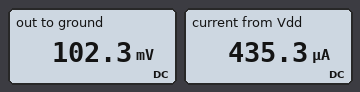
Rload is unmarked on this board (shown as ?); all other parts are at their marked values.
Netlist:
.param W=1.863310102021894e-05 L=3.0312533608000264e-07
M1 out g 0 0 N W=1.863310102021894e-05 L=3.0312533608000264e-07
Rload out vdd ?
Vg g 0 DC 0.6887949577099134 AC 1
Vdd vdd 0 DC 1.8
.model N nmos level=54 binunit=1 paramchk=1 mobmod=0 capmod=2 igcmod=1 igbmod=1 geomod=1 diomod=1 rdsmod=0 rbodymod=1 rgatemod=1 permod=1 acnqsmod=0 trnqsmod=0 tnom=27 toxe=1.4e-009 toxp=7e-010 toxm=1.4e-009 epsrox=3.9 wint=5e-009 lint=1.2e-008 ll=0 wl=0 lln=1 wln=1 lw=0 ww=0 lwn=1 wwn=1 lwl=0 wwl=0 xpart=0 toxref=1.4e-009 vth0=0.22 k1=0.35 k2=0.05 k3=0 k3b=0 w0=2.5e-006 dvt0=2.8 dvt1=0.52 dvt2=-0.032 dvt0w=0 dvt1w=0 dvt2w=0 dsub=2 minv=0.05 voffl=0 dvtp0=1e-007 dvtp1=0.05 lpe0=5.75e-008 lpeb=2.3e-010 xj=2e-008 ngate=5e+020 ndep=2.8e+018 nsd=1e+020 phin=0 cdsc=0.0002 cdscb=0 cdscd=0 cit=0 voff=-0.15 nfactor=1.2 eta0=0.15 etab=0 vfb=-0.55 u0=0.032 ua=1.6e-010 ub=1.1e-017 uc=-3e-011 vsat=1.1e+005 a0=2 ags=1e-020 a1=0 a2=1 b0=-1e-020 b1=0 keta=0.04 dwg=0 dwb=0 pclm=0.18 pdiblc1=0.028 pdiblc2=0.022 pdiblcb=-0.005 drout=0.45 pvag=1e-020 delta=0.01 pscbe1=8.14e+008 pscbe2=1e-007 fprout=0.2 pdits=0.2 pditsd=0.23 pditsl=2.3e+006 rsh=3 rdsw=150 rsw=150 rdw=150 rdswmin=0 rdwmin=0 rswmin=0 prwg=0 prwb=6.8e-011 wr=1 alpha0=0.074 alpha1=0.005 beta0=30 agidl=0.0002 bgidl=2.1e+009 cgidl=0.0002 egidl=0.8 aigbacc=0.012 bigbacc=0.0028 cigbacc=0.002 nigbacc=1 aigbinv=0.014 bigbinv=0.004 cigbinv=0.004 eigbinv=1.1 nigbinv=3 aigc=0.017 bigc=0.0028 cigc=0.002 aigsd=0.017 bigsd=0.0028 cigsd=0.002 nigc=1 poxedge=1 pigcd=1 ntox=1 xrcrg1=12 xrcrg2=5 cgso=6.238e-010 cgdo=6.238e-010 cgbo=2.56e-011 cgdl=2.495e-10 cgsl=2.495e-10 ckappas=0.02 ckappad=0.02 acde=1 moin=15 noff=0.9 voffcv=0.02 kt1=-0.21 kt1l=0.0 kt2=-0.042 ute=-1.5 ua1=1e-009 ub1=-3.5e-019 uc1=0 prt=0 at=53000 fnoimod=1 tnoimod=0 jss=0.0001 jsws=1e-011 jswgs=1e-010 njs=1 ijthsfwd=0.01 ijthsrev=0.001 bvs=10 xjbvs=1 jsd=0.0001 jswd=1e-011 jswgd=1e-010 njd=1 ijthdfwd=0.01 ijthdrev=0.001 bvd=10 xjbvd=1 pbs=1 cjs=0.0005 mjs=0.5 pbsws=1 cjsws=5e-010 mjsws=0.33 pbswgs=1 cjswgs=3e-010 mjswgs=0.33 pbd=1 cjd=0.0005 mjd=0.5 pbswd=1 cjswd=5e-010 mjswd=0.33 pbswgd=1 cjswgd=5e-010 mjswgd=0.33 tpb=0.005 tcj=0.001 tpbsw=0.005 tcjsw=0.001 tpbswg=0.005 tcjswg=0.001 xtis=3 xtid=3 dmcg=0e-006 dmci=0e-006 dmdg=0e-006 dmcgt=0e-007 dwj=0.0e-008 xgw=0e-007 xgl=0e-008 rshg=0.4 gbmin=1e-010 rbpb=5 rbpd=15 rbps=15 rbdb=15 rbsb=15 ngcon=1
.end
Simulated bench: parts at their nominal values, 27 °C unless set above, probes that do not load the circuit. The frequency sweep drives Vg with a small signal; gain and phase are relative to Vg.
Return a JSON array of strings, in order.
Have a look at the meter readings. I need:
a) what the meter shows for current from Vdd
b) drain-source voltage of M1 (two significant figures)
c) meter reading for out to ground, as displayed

["435.3 µA", "100 mV", "102.3 mV"]
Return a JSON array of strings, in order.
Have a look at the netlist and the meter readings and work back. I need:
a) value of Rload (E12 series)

["3.9 kΩ"]
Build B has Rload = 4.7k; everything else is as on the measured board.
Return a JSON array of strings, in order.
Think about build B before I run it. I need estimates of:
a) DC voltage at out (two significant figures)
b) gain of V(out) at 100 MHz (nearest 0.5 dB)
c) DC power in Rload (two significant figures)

["83 mV", "-18.5 dB", "630 µW"]
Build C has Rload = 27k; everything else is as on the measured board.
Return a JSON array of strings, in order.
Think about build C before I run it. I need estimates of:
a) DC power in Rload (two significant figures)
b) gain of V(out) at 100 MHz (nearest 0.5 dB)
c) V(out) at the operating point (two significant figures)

["120 µW", "-34.0 dB", "13 mV"]
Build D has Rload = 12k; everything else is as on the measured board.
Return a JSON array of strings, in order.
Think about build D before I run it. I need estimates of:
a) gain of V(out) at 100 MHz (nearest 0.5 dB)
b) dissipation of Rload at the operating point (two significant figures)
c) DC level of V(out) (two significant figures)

["-29.0 dB", "260 µW", "31 mV"]
